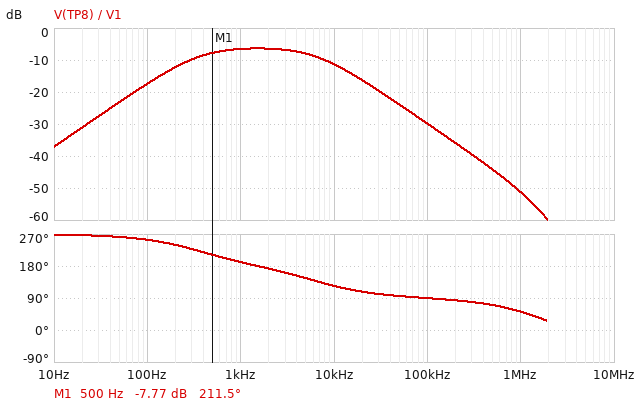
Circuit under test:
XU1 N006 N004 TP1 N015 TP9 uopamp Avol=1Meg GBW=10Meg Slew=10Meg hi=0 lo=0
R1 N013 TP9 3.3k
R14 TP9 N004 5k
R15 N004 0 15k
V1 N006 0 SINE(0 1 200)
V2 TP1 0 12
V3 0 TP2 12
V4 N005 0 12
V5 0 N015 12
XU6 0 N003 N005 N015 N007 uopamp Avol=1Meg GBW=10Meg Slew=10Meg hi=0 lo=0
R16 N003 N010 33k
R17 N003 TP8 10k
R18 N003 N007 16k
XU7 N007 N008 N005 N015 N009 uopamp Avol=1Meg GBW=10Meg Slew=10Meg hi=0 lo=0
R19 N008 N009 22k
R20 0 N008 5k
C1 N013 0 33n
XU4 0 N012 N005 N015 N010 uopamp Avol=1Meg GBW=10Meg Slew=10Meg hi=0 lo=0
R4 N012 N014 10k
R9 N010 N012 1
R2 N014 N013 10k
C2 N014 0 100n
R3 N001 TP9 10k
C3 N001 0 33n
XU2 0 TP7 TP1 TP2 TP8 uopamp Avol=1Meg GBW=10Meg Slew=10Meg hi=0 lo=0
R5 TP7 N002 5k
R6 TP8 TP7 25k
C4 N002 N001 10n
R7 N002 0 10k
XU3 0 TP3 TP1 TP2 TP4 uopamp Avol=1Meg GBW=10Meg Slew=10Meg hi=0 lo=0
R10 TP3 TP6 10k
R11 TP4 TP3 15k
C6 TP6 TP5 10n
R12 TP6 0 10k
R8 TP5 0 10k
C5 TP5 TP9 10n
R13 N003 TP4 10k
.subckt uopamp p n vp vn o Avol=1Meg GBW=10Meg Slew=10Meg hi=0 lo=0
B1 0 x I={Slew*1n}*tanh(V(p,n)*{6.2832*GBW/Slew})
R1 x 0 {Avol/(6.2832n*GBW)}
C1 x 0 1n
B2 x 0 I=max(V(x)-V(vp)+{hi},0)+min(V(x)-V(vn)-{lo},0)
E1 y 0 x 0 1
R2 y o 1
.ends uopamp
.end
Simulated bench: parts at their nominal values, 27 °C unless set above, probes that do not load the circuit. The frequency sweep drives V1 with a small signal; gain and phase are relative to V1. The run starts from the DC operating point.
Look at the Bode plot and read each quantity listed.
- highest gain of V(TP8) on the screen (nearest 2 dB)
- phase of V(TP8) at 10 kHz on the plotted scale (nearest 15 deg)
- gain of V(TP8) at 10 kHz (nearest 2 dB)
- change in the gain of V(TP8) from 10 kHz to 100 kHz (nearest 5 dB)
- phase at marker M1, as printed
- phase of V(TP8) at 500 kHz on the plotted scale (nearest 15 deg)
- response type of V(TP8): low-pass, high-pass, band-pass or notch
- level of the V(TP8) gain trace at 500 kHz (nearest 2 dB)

-6 dB
120 deg
-12 dB
-20 dB
211.5 deg
75 deg
band-pass
-44 dB
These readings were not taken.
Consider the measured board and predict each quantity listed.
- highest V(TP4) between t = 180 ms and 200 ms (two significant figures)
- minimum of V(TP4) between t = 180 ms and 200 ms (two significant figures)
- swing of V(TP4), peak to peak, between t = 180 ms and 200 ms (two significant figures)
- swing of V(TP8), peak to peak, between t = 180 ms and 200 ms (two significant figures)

15 mV
-15 mV
30 mV
490 mV
